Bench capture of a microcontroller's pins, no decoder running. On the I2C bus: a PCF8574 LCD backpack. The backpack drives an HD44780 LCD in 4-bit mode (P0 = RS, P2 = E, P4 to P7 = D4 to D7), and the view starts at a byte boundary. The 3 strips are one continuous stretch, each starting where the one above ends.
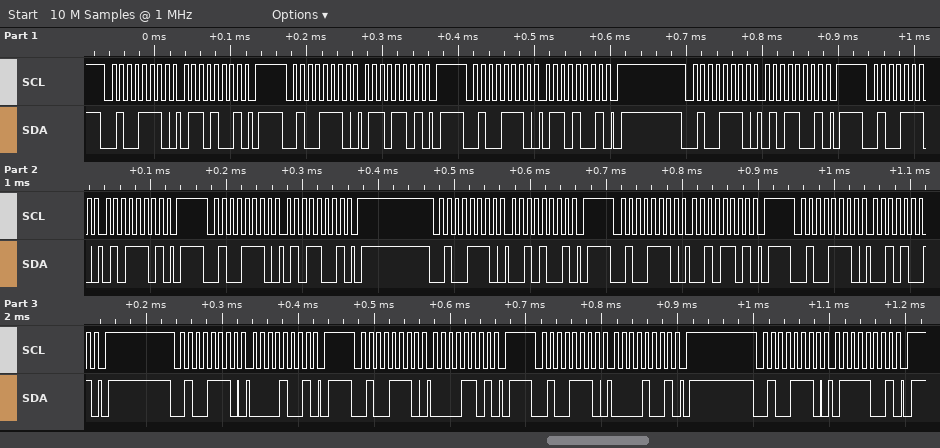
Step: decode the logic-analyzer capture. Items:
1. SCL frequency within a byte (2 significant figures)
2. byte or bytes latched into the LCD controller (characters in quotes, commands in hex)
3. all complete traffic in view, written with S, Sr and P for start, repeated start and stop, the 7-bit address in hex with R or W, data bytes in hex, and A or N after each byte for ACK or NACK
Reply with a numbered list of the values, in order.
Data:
1. 100 kHz
2. 'e' ' '
3. S 27W A 69 A P S 27W A 6D A P S 27W A 69 A P S 27W A 59 A P S 27W A 5D A P S 27W A 59 A P S 27W A 29 A P S 27W A 2D A P S 27W A 29 A P S 27W A 09 A P S 27W A 0D A P S 27W A 09 A P S 27W A 79 A P
